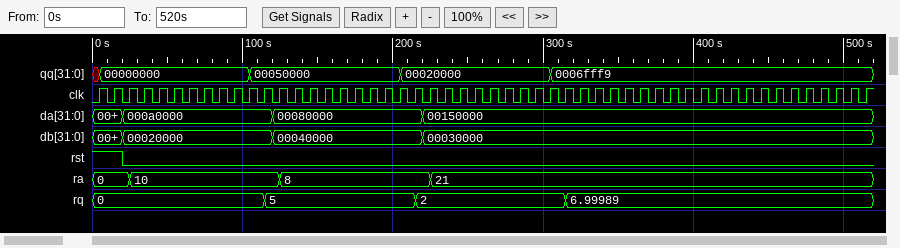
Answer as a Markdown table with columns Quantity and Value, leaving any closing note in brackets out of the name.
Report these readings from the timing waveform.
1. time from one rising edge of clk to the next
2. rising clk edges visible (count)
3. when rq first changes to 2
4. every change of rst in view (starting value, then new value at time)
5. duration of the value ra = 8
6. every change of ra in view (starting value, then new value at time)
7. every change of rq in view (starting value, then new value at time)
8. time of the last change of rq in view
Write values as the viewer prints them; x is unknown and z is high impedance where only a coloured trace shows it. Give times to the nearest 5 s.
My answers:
| Quantity | Value |
|---|---|
| time from one rising edge of clk to the next | 10 s |
| rising clk edges visible | 52 |
| when rq first changes to 2 | 215 s |
| every change of rst in view | 1, 0 at 20 s |
| duration of the value ra = 8 | 100 s |
| every change of ra in view | 0, 10 at 25 s, 8 at 125 s, 21 at 225 s |
| every change of rq in view | 0, 5 at 115 s, 2 at 215 s, 6.99989 at 315 s |
| time of the last change of rq in view | 315 s |
